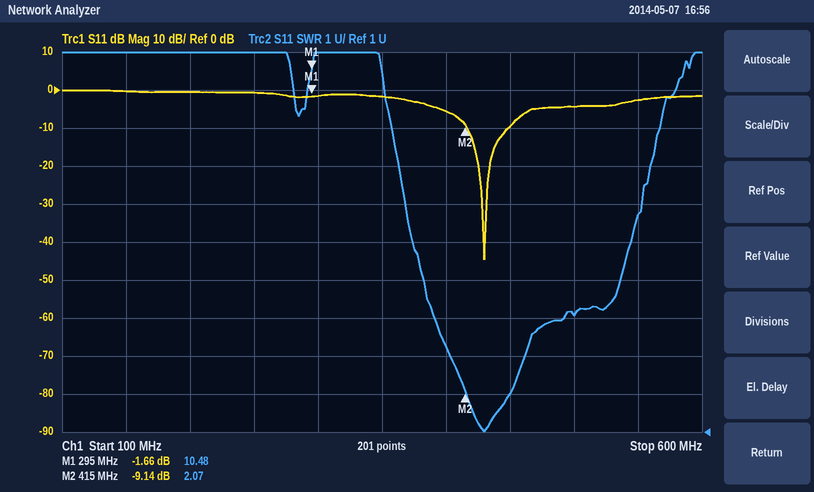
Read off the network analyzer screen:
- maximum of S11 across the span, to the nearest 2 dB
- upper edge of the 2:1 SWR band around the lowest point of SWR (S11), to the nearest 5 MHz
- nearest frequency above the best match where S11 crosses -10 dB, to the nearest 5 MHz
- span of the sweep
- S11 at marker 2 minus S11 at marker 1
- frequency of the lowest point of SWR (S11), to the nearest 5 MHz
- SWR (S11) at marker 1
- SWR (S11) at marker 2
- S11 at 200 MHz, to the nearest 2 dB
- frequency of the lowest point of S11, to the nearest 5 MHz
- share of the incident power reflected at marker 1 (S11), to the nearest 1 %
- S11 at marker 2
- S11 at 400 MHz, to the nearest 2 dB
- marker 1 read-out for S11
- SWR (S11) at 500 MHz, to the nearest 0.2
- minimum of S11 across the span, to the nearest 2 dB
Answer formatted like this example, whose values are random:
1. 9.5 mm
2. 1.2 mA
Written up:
1. 0 dB
2. 450 MHz
3. 450 MHz
4. 500 MHz
5. -7.48 dB
6. 430 MHz
7. 10.48
8. 2.07
9. 0 dB
10. 430 MHz
11. 68 %
12. -9.14 dB
13. -6 dB
14. -1.66 dB
15. 4.0
16. -44 dB
